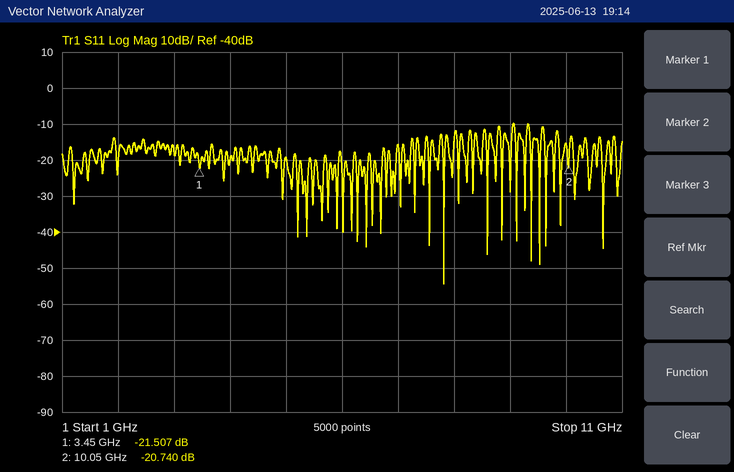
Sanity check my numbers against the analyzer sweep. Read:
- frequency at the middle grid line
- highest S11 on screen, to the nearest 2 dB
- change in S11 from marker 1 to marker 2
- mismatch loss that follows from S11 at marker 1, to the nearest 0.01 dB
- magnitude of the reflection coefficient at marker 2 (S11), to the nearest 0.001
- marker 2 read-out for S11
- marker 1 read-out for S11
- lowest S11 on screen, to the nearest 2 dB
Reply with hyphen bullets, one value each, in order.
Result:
- 6 GHz
- -10 dB
- 0.767 dB
- 0.03 dB
- 0.092
- -20.740 dB
- -21.507 dB
- -54 dB
